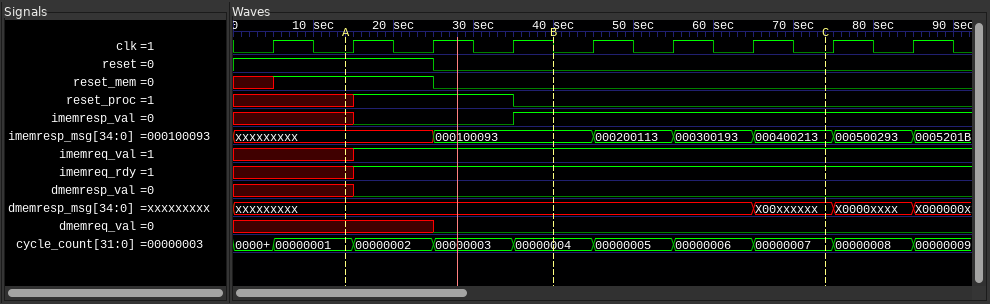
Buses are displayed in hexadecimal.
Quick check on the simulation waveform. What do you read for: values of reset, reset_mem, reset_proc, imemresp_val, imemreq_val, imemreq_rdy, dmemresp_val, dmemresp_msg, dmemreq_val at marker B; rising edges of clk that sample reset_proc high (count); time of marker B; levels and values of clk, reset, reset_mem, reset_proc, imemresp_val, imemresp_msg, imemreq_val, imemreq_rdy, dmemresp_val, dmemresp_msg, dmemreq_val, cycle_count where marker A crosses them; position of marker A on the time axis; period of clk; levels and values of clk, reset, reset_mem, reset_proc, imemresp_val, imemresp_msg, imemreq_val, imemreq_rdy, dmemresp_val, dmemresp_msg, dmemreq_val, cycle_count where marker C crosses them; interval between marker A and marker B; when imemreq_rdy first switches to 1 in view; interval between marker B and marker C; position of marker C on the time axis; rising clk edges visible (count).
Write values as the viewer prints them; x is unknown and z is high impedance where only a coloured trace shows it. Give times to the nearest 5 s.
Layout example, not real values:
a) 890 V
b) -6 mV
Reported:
a) reset=0, reset_mem=0, reset_proc=0, imemresp_val=1, imemreq_val=1, imemreq_rdy=1, dmemresp_val=0, dmemresp_msg=xxxxxxxxx, dmemreq_val=0
b) 2
c) 40 s
d) clk=0, reset=1, reset_mem=1, reset_proc=x, imemresp_val=x, imemresp_msg=xxxxxxxxx, imemreq_val=x, imemreq_rdy=x, dmemresp_val=x, dmemresp_msg=xxxxxxxxx, dmemreq_val=x, cycle_count=00000001
e) 15 s
f) 10 s
g) clk=0, reset=0, reset_mem=0, reset_proc=0, imemresp_val=1, imemresp_msg=000400213, imemreq_val=1, imemreq_rdy=1, dmemresp_val=0, dmemresp_msg=X00xxxxxx, dmemreq_val=0, cycle_count=00000007
h) 25 s
i) 15 s
j) 35 s
k) 75 s
l) 9
